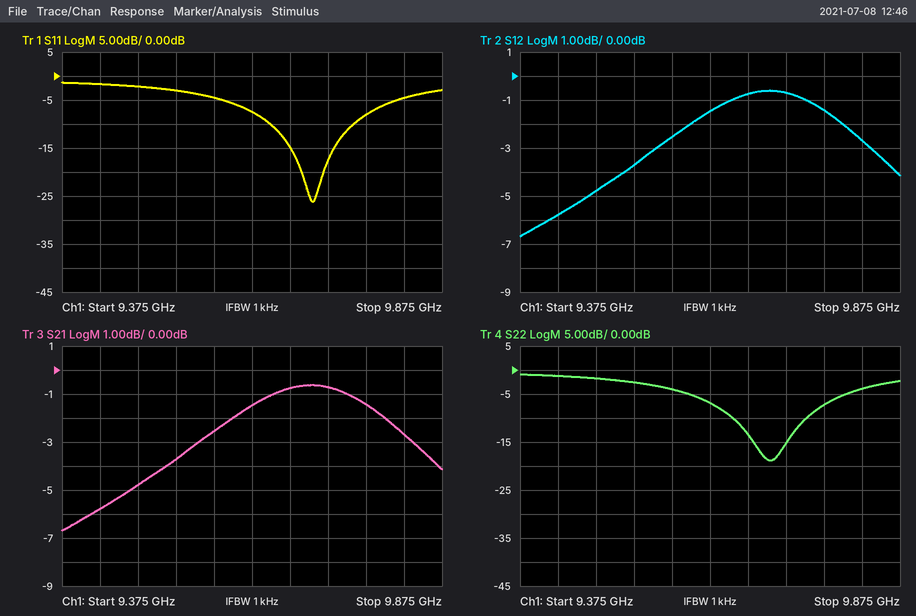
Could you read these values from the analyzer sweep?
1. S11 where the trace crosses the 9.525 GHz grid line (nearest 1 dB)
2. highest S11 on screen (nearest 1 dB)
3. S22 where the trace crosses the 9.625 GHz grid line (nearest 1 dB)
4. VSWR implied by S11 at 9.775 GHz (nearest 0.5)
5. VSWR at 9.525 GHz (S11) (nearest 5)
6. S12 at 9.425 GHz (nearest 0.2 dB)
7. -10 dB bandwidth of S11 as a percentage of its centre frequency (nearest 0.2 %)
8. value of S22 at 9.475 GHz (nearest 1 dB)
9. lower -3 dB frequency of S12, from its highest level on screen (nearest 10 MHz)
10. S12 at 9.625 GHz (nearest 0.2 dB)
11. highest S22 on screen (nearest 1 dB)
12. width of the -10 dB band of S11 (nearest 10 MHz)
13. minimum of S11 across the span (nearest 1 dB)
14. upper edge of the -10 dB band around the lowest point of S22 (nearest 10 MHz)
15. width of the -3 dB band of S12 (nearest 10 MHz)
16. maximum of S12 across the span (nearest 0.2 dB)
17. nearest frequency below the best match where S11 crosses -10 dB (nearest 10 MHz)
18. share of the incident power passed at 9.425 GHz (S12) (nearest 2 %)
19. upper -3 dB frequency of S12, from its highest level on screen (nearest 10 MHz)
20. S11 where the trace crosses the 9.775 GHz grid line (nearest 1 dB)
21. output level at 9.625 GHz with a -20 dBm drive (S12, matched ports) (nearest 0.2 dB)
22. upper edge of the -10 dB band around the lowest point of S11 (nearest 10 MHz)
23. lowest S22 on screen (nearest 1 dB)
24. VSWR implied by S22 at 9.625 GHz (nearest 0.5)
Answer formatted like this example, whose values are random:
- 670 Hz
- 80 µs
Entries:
- -3 dB
- -1 dB
- -7 dB
- 2.5
- 5
- -5.8 dB
- 1.2 %
- -2 dB
- 9.53 GHz
- -1.4 dB
- -1 dB
- 110 MHz
- -26 dB
- 9.75 GHz
- 330 MHz
- -0.6 dB
- 9.65 GHz
- 26 %
- 9.86 GHz
- -8 dB
- -21.4 dBm
- 9.76 GHz
- -19 dB
- 2.5
